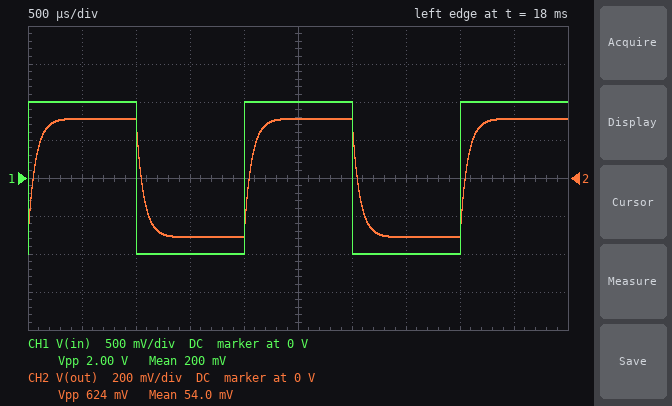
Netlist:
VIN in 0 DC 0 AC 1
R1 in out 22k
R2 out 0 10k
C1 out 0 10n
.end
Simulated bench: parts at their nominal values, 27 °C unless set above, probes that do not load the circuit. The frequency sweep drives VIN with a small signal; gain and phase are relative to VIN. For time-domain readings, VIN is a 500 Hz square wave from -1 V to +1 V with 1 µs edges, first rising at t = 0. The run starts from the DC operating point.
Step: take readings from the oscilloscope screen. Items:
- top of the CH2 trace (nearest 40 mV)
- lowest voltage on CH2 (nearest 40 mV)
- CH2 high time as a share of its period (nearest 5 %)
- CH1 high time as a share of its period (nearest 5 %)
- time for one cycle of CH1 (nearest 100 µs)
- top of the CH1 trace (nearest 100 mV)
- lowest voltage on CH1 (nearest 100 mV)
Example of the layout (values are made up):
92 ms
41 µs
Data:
320 mV
-320 mV
50 %
50 %
2.0 ms
1.0 V
-1.0 V
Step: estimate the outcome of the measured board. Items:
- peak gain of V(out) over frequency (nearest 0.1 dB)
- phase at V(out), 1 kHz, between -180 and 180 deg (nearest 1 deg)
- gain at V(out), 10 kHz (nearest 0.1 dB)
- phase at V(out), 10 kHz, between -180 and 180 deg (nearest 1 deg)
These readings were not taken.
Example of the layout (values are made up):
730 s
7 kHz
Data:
-10.1 dB
-23 deg
-23.0 dB
-77 deg
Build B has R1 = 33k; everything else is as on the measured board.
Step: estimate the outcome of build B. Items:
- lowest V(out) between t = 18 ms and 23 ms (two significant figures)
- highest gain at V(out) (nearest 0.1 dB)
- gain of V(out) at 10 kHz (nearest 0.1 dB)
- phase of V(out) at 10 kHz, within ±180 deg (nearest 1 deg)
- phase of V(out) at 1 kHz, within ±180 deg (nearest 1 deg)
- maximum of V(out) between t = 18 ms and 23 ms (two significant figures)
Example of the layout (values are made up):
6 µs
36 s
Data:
-230 mV
-12.7 dB
-26.5 dB
-78 deg
-26 deg
230 mV
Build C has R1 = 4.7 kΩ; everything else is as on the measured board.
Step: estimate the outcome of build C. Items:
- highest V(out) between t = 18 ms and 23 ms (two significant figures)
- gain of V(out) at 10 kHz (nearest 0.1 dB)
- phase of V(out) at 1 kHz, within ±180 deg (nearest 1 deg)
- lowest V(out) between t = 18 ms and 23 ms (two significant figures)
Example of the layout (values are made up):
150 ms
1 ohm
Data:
680 mV
-10.4 dB
-11 deg
-680 mV
